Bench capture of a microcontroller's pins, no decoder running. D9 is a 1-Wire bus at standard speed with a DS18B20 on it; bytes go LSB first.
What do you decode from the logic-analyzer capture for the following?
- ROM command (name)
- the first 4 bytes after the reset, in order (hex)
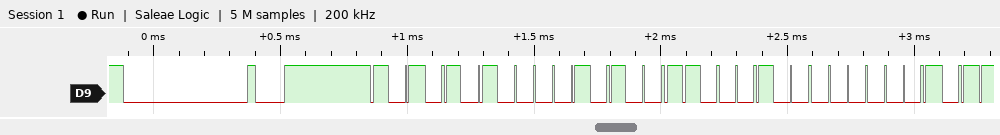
Match ROM
55 28 23 40
